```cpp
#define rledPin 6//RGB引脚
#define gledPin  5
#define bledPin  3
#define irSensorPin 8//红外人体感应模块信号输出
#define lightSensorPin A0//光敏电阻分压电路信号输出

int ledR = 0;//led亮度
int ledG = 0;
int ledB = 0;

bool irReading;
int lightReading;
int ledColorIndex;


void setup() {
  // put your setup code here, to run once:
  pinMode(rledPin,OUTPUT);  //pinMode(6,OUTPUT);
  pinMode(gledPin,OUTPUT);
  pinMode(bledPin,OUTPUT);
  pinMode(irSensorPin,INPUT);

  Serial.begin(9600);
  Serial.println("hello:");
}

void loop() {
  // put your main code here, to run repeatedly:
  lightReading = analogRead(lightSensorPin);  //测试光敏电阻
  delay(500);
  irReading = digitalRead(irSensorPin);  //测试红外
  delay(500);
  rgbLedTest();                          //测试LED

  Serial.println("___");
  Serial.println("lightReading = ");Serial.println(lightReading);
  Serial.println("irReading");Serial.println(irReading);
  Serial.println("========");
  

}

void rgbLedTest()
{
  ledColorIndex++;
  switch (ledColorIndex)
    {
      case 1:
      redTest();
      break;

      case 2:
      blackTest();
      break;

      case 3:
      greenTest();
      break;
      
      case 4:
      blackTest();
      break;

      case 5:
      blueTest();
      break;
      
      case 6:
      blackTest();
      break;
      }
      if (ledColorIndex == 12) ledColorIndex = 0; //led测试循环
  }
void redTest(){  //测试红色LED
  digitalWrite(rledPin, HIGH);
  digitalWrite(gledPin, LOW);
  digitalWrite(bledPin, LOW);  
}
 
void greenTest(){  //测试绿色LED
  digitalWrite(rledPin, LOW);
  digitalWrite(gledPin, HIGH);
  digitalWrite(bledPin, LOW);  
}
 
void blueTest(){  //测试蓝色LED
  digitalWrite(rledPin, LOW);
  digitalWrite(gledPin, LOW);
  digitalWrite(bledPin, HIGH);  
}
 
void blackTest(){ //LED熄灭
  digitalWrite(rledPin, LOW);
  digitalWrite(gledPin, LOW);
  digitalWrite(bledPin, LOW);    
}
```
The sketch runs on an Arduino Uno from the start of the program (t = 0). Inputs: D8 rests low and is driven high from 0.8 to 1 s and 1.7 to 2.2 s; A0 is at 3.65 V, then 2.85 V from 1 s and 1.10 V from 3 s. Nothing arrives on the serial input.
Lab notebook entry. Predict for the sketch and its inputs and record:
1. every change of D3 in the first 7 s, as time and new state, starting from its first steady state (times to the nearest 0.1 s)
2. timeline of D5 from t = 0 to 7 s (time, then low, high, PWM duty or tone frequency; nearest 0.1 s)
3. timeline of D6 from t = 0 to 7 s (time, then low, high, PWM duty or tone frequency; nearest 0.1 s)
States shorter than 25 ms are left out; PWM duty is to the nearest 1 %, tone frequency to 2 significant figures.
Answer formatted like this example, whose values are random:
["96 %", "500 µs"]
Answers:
["0 s low; 5 s high; 6 s low", "0 s low; 3 s high; 4 s low", "0 s low; 1 s high; 2 s low"]
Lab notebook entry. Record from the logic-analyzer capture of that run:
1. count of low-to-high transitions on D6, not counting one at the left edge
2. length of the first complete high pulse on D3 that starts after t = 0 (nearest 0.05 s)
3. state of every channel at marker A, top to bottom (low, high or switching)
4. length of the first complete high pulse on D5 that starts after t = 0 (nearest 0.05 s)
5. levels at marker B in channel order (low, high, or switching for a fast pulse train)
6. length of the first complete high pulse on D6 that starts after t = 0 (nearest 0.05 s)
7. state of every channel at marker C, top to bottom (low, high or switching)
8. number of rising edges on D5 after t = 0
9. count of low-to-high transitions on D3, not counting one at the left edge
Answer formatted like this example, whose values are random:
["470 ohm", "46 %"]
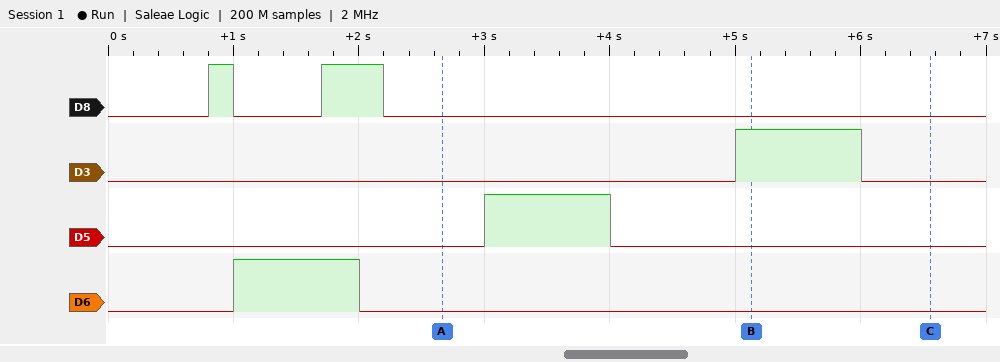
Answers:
["1", "1.00 s", "D8 low, D3 low, D5 low, D6 low", "1.00 s", "D8 low, D3 high, D5 low, D6 low", "1.00 s", "D8 low, D3 low, D5 low, D6 low", "1", "1"]
